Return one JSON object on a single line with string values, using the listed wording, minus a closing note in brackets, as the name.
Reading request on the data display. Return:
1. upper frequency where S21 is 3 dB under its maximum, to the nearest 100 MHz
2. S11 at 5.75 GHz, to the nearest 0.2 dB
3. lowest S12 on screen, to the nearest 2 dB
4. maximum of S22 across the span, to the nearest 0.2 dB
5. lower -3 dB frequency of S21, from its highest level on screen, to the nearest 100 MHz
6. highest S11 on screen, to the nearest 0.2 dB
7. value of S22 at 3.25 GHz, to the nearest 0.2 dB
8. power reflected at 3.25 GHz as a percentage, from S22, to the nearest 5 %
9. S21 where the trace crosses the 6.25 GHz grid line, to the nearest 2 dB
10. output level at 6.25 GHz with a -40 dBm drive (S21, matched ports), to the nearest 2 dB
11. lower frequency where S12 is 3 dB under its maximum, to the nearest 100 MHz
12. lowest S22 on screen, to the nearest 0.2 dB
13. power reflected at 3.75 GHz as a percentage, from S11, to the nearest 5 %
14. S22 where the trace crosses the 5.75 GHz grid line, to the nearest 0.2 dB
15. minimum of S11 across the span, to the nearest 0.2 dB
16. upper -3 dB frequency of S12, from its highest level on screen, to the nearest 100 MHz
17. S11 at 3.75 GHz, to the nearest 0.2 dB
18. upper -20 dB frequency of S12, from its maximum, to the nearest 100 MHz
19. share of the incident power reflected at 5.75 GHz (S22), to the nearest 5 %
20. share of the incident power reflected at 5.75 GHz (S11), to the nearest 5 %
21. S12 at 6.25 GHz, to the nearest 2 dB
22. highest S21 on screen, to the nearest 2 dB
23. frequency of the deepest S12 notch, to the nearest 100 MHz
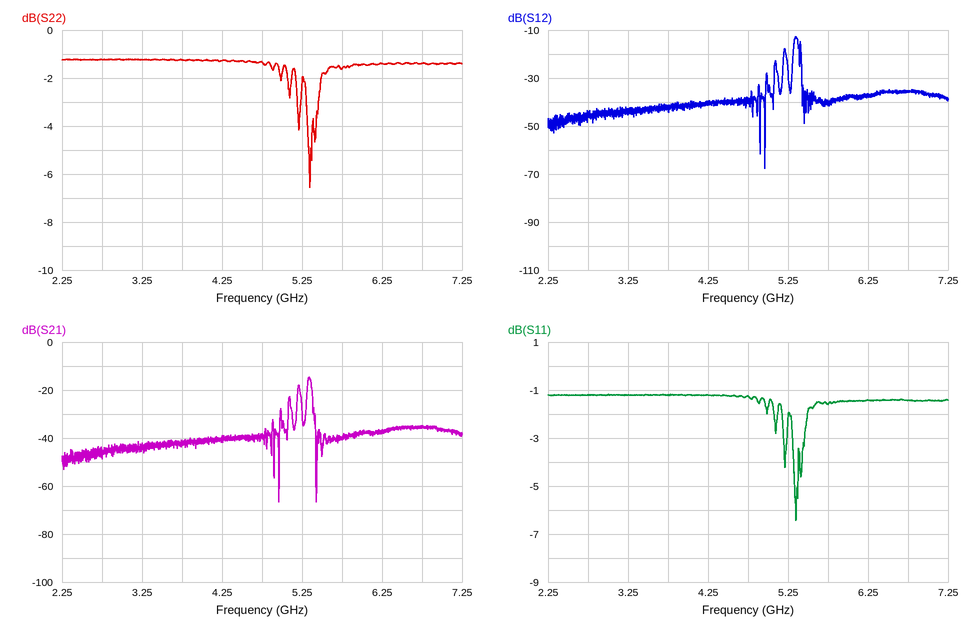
{"upper frequency where S21 is 3 dB under its maximum, to the nearest 100 MHz": "5.4 GHz", "S11 at 5.75 GHz, to the nearest 0.2 dB": "-1.6 dB", "lowest S12 on screen, to the nearest 2 dB": "-68 dB", "maximum of S22 across the span, to the nearest 0.2 dB": "-1.2 dB", "lower -3 dB frequency of S21, from its highest level on screen, to the nearest 100 MHz": "5.3 GHz", "highest S11 on screen, to the nearest 0.2 dB": "-1.2 dB", "value of S22 at 3.25 GHz, to the nearest 0.2 dB": "-1.2 dB", "power reflected at 3.25 GHz as a percentage, from S22, to the nearest 5 %": "75 %", "S21 where the trace crosses the 6.25 GHz grid line, to the nearest 2 dB": "-38 dB", "output level at 6.25 GHz with a -40 dBm drive (S21, matched ports), to the nearest 2 dB": "-78 dBm", "lower frequency where S12 is 3 dB under its maximum, to the nearest 100 MHz": "5.3 GHz", "lowest S22 on screen, to the nearest 0.2 dB": "-6.6 dB", "power reflected at 3.75 GHz as a percentage, from S11, to the nearest 5 %": "75 %", "S22 where the trace crosses the 5.75 GHz grid line, to the nearest 0.2 dB": "-1.6 dB", "minimum of S11 across the span, to the nearest 0.2 dB": "-6.4 dB", "upper -3 dB frequency of S12, from its highest level on screen, to the nearest 100 MHz": "5.4 GHz", "S11 at 3.75 GHz, to the nearest 0.2 dB": "-1.2 dB", "upper -20 dB frequency of S12, from its maximum, to the nearest 100 MHz": "5.4 GHz", "share of the incident power reflected at 5.75 GHz (S22), to the nearest 5 %": "70 %", "share of the incident power reflected at 5.75 GHz (S11), to the nearest 5 %": "70 %", "S12 at 6.25 GHz, to the nearest 2 dB": "-38 dB", "highest S21 on screen, to the nearest 2 dB": "-14 dB", "frequency of the deepest S12 notch, to the nearest 100 MHz": "5.0 GHz"}
